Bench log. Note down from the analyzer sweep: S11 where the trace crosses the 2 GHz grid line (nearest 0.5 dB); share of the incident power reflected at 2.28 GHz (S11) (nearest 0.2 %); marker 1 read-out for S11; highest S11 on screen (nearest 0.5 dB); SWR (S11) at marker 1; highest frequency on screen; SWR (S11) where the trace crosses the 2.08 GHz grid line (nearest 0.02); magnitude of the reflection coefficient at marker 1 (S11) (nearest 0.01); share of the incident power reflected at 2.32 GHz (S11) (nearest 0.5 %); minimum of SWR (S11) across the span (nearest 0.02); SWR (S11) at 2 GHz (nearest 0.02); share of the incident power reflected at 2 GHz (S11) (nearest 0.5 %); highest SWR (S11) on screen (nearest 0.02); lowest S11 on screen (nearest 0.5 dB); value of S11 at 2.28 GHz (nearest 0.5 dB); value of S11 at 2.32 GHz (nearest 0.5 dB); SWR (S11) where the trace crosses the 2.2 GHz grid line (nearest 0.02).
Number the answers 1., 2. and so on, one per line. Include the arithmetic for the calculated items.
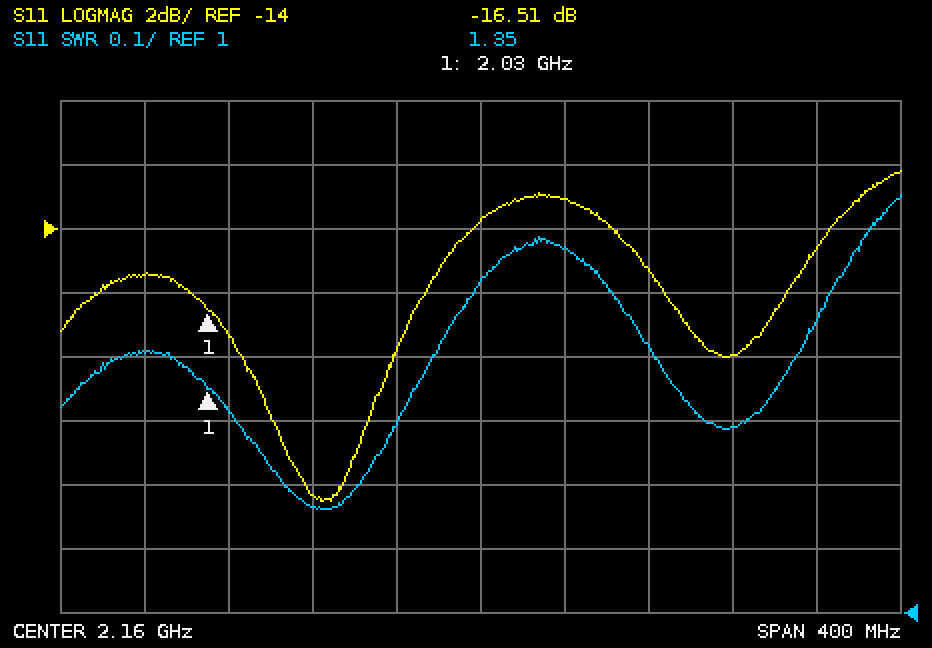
1. -15.5 dB
2. 10^(-18/10) ≈ 1.6 %
3. -16.51 dB
4. -12.0 dB
5. 1.35
6. 2.36 GHz
7. 1.16
8. 10^(-16.51/20) ≈ 0.15
9. 10^(-14.5/10) ≈ 3.5 %
10. 1.16
11. 1.40
12. 10^(-15.5/10) ≈ 2.82 %, so 3.0 % to the nearest 0.5 %
13. 1.66
14. -22.5 dB
15. -18.0 dB
16. -14.5 dB
17. 1.58
